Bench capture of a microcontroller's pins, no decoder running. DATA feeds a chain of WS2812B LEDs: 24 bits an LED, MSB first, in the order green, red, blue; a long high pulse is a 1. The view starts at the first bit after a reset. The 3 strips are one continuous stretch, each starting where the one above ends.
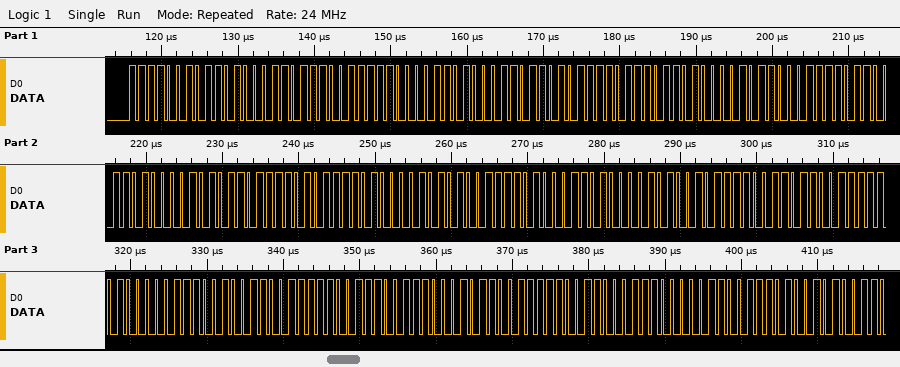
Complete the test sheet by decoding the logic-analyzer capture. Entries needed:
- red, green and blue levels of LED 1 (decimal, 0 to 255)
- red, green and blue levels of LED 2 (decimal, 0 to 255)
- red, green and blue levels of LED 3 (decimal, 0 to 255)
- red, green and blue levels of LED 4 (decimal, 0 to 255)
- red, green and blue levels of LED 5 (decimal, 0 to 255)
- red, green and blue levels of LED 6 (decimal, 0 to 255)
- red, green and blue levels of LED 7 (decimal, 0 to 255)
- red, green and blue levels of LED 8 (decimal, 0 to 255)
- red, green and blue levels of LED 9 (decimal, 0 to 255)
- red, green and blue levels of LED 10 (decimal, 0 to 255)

209, 242, 185
209, 240, 181
208, 238, 177
208, 236, 173
208, 235, 169
208, 232, 165
207, 230, 160
207, 228, 156
207, 226, 152
206, 224, 148
